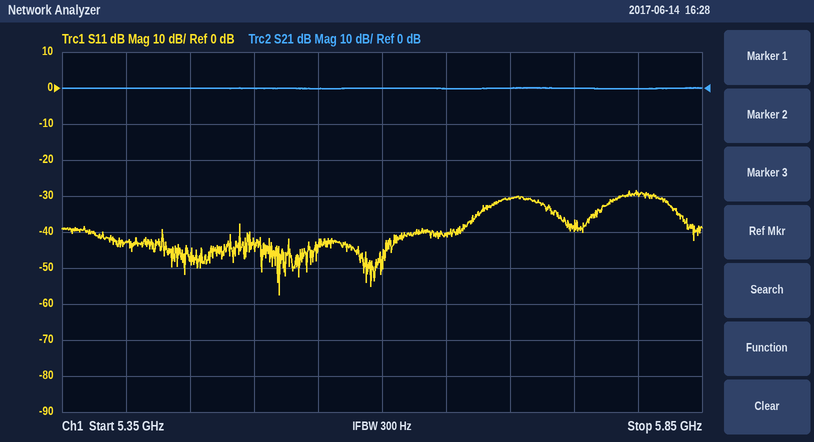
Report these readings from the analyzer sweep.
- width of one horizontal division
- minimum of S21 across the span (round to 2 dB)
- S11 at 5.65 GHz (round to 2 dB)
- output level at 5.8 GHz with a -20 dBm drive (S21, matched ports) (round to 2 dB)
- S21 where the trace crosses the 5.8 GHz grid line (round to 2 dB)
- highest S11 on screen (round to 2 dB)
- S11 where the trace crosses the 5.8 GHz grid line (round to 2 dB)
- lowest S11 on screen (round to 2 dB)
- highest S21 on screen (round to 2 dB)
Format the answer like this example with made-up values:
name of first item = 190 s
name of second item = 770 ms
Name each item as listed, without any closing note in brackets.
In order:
width of one horizontal division = 50 MHz
minimum of S21 across the span = 0 dB
S11 at 5.65 GHz = -40 dB
output level at 5.8 GHz with a -20 dBm drive (S21, matched ports) = -20 dBm
S21 where the trace crosses the 5.8 GHz grid line = 0 dB
highest S11 on screen = -28 dB
S11 where the trace crosses the 5.8 GHz grid line = -30 dB
lowest S11 on screen = -58 dB
highest S21 on screen = 0 dB
